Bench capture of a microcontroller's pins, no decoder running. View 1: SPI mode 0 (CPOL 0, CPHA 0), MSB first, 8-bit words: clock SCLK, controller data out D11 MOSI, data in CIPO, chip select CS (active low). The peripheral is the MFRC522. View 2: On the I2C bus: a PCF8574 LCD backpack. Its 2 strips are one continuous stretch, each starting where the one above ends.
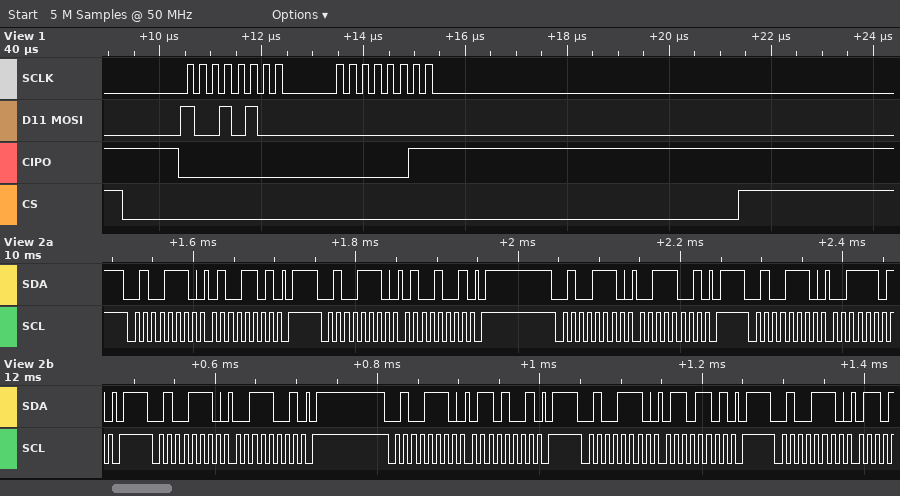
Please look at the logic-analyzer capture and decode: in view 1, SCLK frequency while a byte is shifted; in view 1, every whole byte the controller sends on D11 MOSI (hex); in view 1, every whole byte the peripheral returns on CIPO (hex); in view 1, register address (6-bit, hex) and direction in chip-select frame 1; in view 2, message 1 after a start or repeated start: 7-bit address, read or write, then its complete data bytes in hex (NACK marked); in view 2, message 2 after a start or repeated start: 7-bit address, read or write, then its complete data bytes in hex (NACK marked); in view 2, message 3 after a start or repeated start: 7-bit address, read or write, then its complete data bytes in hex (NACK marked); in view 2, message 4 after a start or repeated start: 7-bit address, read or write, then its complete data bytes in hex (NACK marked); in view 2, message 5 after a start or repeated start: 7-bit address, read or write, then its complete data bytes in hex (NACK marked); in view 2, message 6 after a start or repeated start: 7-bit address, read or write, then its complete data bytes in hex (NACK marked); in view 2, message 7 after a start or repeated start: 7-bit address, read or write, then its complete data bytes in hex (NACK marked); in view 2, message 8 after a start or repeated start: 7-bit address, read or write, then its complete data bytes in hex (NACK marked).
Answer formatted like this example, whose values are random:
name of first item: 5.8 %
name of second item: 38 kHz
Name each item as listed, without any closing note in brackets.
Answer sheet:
in view 1, SCLK frequency while a byte is shifted: 4 MHz
in view 1, every whole byte the controller sends on D11 MOSI: 0x94 0x00
in view 1, every whole byte the peripheral returns on CIPO: 0x00 0x03
in view 1, register address (6-bit, hex) and direction in chip-select frame 1: 0x0A read
in view 2, message 1 after a start or repeated start: 7-bit address, read or write, then its complete data bytes in hex: 0x27 write: 4D
in view 2, message 2 after a start or repeated start: 7-bit address, read or write, then its complete data bytes in hex: 0x27 write: 49
in view 2, message 3 after a start or repeated start: 7-bit address, read or write, then its complete data bytes in hex: 0x27 write: 39
in view 2, message 4 after a start or repeated start: 7-bit address, read or write, then its complete data bytes in hex: 0x27 write: 3D
in view 2, message 5 after a start or repeated start: 7-bit address, read or write, then its complete data bytes in hex: 0x27 write: 39
in view 2, message 6 after a start or repeated start: 7-bit address, read or write, then its complete data bytes in hex: 0x27 write: 69
in view 2, message 7 after a start or repeated start: 7-bit address, read or write, then its complete data bytes in hex: 0x27 write: 6D
in view 2, message 8 after a start or repeated start: 7-bit address, read or write, then its complete data bytes in hex: 0x27 write
